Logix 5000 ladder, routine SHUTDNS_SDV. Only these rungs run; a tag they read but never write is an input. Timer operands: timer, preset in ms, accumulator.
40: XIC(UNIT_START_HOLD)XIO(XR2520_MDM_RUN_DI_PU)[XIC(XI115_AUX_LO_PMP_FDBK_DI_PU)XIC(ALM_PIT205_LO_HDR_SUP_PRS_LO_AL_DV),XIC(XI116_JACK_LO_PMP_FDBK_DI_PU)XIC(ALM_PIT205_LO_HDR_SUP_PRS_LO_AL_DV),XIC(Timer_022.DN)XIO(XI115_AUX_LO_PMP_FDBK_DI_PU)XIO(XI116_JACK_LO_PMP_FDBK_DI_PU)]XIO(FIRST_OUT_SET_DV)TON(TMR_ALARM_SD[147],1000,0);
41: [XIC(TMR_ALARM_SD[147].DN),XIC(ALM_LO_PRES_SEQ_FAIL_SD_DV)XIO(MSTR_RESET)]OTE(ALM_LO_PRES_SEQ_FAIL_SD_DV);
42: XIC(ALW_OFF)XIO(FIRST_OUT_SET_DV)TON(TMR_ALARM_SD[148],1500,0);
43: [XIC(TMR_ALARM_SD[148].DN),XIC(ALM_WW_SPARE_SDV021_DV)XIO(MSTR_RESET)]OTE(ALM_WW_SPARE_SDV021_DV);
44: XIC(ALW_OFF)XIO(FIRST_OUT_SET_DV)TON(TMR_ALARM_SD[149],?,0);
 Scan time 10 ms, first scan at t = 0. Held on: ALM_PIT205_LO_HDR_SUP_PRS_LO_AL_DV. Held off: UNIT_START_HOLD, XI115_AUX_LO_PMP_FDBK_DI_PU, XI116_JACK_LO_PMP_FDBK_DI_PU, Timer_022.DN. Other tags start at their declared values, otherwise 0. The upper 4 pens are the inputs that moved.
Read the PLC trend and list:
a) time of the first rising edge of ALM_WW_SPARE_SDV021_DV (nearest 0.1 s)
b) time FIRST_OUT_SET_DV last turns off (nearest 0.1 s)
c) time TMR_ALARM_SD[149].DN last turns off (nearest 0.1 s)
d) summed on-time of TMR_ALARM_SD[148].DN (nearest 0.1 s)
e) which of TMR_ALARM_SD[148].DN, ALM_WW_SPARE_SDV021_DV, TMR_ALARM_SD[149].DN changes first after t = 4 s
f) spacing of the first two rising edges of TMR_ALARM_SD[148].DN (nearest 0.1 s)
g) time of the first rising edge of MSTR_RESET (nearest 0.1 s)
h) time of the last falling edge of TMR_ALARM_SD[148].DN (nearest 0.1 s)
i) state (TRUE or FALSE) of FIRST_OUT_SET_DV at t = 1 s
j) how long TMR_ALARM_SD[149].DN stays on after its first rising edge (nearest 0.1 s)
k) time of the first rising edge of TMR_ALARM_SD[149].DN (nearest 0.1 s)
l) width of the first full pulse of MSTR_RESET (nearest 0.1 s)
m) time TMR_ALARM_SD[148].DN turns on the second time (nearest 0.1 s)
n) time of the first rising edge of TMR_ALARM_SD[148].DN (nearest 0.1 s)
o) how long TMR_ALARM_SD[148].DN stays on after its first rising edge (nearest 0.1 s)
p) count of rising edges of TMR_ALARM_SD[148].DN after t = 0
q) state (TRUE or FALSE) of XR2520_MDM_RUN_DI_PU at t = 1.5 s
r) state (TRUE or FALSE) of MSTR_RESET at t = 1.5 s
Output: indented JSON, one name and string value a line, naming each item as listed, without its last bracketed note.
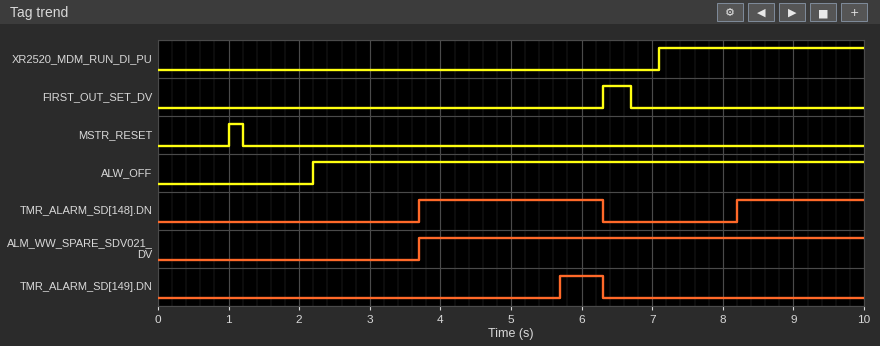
{
  "time of the first rising edge of ALM_WW_SPARE_SDV021_DV": "3.7 s",
  "time FIRST_OUT_SET_DV last turns off": "6.7 s",
  "time TMR_ALARM_SD[149].DN last turns off": "6.3 s",
  "summed on-time of TMR_ALARM_SD[148].DN": "4.4 s",
  "which of TMR_ALARM_SD[148].DN, ALM_WW_SPARE_SDV021_DV, TMR_ALARM_SD[149].DN changes first after t = 4 s": "TMR_ALARM_SD[149].DN",
  "spacing of the first two rising edges of TMR_ALARM_SD[148].DN": "4.5 s",
  "time of the first rising edge of MSTR_RESET": "1.0 s",
  "time of the last falling edge of TMR_ALARM_SD[148].DN": "6.3 s",
  "state (TRUE or FALSE) of FIRST_OUT_SET_DV at t = 1 s": "FALSE",
  "how long TMR_ALARM_SD[149].DN stays on after its first rising edge": "0.6 s",
  "time of the first rising edge of TMR_ALARM_SD[149].DN": "5.7 s",
  "width of the first full pulse of MSTR_RESET": "0.2 s",
  "time TMR_ALARM_SD[148].DN turns on the second time": "8.2 s",
  "time of the first rising edge of TMR_ALARM_SD[148].DN": "3.7 s",
  "how long TMR_ALARM_SD[148].DN stays on after its first rising edge": "2.6 s",
  "count of rising edges of TMR_ALARM_SD[148].DN after t = 0": "2",
  "state (TRUE or FALSE) of XR2520_MDM_RUN_DI_PU at t = 1.5 s": "FALSE",
  "state (TRUE or FALSE) of MSTR_RESET at t = 1.5 s": "FALSE"
}
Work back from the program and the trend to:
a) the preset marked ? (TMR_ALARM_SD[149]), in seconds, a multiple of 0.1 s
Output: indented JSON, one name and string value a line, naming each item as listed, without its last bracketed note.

{
  "the preset marked ? (TMR_ALARM_SD[149]), in seconds, a multiple of 0.1 s": "3.5 s"
}
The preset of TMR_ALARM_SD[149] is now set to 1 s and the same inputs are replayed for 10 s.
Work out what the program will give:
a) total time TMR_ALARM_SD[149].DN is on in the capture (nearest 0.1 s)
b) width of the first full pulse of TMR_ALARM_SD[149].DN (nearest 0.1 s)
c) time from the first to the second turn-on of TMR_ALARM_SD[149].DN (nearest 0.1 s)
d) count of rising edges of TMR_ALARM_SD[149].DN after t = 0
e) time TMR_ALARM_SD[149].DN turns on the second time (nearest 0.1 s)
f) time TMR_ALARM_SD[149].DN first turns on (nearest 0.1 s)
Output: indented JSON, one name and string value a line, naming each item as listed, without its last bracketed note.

{
  "total time TMR_ALARM_SD[149].DN is on in the capture": "5.4 s",
  "width of the first full pulse of TMR_ALARM_SD[149].DN": "3.1 s",
  "time from the first to the second turn-on of TMR_ALARM_SD[149].DN": "4.5 s",
  "count of rising edges of TMR_ALARM_SD[149].DN after t = 0": "2",
  "time TMR_ALARM_SD[149].DN turns on the second time": "7.7 s",
  "time TMR_ALARM_SD[149].DN first turns on": "3.2 s"
}
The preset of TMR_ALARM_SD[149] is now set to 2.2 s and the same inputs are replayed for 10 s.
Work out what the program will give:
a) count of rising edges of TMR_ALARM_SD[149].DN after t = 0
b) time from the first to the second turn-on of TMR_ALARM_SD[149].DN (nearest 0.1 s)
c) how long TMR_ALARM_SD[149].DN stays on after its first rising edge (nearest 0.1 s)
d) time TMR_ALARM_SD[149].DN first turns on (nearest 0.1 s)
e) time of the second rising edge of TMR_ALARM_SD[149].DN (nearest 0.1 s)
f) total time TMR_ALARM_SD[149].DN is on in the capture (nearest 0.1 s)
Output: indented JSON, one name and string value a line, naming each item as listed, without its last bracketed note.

{
  "count of rising edges of TMR_ALARM_SD[149].DN after t = 0": "2",
  "time from the first to the second turn-on of TMR_ALARM_SD[149].DN": "4.5 s",
  "how long TMR_ALARM_SD[149].DN stays on after its first rising edge": "1.9 s",
  "time TMR_ALARM_SD[149].DN first turns on": "4.4 s",
  "time of the second rising edge of TMR_ALARM_SD[149].DN": "8.9 s",
  "total time TMR_ALARM_SD[149].DN is on in the capture": "3.0 s"
}
